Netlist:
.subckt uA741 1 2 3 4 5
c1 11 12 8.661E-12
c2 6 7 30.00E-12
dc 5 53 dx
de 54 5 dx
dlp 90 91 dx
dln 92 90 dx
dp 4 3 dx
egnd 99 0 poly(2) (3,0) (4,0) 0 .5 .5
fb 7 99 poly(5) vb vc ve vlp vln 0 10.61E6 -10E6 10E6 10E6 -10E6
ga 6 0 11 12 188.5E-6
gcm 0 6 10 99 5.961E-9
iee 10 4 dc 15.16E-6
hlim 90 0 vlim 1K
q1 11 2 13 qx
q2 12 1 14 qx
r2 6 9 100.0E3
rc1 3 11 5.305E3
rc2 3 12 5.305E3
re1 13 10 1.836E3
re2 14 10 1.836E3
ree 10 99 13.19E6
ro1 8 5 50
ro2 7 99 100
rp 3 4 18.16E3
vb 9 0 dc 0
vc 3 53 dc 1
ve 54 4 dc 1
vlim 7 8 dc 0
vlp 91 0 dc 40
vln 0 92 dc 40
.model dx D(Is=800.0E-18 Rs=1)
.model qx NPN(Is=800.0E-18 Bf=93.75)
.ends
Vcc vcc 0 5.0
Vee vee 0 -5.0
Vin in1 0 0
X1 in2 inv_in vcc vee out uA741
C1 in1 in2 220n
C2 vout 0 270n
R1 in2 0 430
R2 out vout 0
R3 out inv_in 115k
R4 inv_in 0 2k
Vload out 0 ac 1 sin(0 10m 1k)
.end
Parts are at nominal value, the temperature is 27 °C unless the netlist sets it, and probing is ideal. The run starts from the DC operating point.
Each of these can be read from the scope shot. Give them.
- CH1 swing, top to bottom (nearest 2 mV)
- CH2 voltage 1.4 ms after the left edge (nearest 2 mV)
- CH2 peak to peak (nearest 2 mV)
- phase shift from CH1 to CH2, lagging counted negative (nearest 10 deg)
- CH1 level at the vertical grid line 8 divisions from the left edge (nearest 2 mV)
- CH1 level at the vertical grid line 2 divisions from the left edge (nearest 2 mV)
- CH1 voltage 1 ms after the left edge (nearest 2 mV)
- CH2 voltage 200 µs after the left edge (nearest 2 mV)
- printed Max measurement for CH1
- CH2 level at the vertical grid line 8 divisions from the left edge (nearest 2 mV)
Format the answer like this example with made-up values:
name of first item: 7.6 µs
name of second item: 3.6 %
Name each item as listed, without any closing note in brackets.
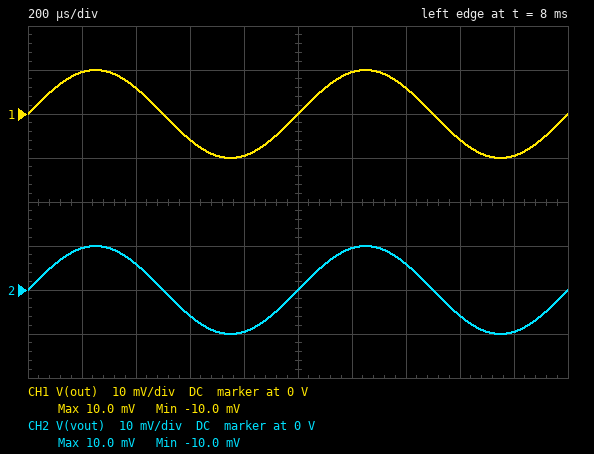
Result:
CH1 swing, top to bottom: 20 mV
CH2 voltage 1.4 ms after the left edge: 6 mV
CH2 peak to peak: 20 mV
phase shift from CH1 to CH2, lagging counted negative: 0 deg
CH1 level at the vertical grid line 8 divisions from the left edge: -6 mV
CH1 level at the vertical grid line 2 divisions from the left edge: 6 mV
CH1 voltage 1 ms after the left edge: 0 V
CH2 voltage 200 µs after the left edge: 10 mV
printed Max measurement for CH1: 10.0 mV
CH2 level at the vertical grid line 8 divisions from the left edge: -6 mV
